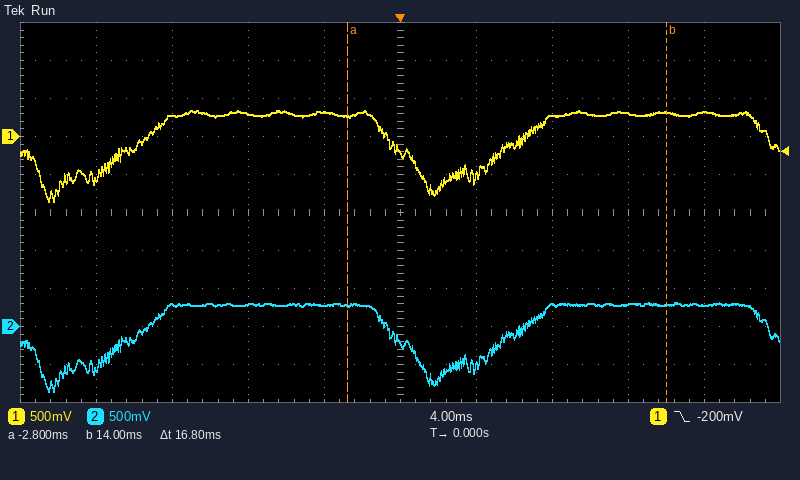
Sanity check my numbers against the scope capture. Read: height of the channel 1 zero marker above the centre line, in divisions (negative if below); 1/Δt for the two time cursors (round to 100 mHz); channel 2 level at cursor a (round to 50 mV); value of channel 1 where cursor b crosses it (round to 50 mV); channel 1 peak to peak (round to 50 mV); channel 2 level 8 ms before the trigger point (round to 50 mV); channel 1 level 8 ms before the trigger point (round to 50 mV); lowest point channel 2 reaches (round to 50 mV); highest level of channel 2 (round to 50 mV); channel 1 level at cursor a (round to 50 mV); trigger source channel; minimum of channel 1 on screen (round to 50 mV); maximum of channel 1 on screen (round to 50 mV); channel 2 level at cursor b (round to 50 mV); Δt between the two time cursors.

+2.0 div
59.5 Hz
300 mV
300 mV
1.20 V
300 mV
300 mV
-850 mV
300 mV
250 mV
channel 1
-850 mV
350 mV
300 mV
16.8 ms
